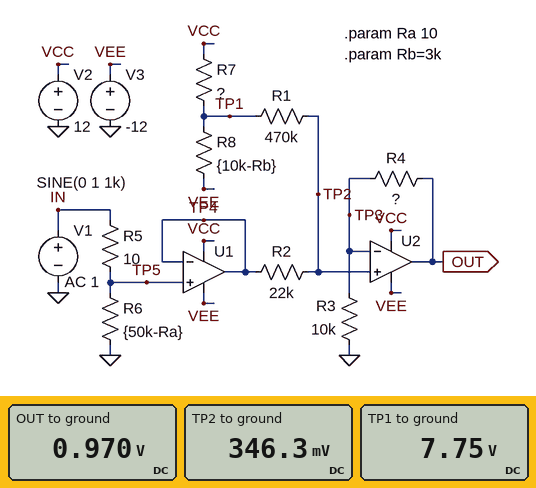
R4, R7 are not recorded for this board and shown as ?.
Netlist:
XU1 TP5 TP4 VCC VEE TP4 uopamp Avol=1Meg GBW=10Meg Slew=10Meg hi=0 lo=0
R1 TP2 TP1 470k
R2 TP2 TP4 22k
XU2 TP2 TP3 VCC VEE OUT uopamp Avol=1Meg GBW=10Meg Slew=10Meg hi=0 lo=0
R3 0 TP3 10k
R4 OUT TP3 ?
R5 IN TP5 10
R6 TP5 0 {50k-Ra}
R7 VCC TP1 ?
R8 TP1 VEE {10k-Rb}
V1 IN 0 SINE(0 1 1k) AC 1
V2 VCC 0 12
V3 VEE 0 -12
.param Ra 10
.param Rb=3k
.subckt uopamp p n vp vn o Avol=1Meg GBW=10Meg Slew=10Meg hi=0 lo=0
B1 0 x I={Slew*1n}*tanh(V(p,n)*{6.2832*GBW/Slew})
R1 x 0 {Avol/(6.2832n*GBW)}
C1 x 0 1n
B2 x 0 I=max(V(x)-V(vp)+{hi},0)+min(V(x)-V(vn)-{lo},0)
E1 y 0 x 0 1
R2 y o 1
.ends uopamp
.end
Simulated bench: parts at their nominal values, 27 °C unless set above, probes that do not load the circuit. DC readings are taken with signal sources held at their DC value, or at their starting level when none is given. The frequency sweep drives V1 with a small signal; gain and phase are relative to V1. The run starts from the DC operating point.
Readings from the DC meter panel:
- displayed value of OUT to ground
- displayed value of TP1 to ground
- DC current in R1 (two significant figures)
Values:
0.970 V
7.75 V
16 µA
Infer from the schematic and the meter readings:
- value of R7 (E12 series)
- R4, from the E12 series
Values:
1.5 kΩ
18 kΩ
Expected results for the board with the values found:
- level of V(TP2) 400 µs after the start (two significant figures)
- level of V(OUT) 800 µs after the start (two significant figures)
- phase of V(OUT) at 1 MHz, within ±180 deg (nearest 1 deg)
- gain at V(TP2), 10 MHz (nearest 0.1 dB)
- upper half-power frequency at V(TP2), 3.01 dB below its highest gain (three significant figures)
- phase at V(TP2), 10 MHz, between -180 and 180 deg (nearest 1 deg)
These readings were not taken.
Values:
910 mV
-1.6 V
-21 deg
-3.4 dB
10.0 MHz
-45 deg
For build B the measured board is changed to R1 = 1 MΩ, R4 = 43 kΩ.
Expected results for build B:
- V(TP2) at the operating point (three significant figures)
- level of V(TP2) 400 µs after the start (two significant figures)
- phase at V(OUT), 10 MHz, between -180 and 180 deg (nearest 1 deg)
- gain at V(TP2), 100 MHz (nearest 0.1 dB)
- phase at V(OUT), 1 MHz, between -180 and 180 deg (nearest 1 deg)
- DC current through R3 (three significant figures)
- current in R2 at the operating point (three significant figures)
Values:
167 mV
740 mV
-124 deg
-20.2 dB
-34 deg
16.7 µA
7.59 µA
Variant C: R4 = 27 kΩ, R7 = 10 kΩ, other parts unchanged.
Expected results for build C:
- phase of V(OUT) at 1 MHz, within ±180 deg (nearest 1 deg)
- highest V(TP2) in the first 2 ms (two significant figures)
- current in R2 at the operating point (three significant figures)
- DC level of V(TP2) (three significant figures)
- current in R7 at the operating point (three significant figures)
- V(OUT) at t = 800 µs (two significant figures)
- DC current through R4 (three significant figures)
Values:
-26 deg
860 mV
4.27 µA
-93.9 mV
1.41 mA
-3.7 V
9.39 µA
